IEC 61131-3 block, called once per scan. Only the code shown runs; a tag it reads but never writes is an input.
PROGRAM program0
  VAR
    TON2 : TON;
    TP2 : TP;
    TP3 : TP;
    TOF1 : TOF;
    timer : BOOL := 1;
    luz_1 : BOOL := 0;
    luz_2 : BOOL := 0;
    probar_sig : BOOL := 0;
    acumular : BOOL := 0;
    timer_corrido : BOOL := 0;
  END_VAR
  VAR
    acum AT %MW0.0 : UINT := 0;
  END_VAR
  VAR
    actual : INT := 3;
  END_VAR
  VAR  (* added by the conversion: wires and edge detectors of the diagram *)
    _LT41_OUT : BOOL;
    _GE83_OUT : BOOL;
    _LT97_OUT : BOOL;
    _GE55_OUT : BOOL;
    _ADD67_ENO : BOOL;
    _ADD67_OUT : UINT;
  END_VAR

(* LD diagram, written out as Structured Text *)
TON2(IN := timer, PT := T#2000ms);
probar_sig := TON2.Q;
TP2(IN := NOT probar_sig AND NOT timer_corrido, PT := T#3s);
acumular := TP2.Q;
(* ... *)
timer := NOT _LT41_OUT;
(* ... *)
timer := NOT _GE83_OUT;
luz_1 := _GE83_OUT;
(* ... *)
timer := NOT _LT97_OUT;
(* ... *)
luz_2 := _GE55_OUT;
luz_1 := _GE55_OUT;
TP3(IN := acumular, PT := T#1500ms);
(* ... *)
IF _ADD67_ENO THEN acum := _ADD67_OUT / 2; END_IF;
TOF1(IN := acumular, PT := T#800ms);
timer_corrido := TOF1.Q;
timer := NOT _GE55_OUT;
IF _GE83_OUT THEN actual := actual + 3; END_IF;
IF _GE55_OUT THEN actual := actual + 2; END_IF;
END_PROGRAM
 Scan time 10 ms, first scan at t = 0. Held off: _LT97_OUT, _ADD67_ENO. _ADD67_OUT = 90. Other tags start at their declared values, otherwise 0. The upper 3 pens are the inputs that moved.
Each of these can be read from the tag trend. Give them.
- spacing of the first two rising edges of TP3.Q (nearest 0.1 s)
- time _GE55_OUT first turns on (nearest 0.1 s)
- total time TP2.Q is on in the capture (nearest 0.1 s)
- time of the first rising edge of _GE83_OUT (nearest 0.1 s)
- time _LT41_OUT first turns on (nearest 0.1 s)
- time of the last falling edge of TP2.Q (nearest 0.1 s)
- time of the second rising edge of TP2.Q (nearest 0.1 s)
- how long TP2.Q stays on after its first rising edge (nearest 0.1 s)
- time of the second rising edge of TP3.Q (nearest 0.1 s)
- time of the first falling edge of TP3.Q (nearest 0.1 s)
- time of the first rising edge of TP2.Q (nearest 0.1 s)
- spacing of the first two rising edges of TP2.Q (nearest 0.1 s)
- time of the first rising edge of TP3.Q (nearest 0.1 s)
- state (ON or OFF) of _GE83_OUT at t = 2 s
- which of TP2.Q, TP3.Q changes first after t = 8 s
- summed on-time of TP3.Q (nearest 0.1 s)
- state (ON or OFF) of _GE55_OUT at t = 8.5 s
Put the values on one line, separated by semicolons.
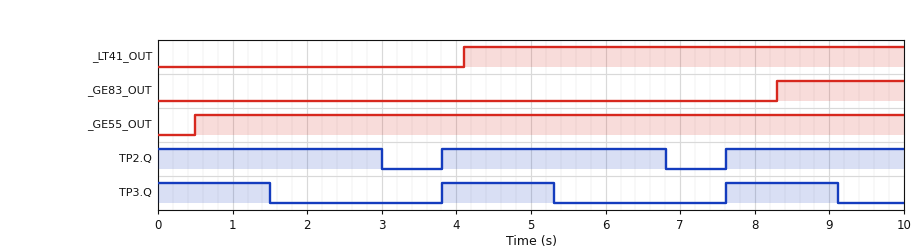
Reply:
3.8 s; 0.5 s; 8.4 s; 8.3 s; 4.1 s; 6.8 s; 7.6 s; 3.0 s; 7.6 s; 1.5 s; 3.8 s; 3.8 s; 3.8 s; OFF; TP3.Q; 4.5 s; ON
